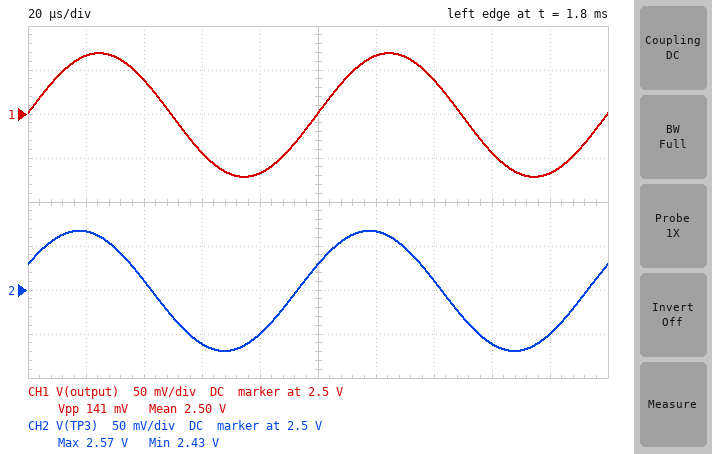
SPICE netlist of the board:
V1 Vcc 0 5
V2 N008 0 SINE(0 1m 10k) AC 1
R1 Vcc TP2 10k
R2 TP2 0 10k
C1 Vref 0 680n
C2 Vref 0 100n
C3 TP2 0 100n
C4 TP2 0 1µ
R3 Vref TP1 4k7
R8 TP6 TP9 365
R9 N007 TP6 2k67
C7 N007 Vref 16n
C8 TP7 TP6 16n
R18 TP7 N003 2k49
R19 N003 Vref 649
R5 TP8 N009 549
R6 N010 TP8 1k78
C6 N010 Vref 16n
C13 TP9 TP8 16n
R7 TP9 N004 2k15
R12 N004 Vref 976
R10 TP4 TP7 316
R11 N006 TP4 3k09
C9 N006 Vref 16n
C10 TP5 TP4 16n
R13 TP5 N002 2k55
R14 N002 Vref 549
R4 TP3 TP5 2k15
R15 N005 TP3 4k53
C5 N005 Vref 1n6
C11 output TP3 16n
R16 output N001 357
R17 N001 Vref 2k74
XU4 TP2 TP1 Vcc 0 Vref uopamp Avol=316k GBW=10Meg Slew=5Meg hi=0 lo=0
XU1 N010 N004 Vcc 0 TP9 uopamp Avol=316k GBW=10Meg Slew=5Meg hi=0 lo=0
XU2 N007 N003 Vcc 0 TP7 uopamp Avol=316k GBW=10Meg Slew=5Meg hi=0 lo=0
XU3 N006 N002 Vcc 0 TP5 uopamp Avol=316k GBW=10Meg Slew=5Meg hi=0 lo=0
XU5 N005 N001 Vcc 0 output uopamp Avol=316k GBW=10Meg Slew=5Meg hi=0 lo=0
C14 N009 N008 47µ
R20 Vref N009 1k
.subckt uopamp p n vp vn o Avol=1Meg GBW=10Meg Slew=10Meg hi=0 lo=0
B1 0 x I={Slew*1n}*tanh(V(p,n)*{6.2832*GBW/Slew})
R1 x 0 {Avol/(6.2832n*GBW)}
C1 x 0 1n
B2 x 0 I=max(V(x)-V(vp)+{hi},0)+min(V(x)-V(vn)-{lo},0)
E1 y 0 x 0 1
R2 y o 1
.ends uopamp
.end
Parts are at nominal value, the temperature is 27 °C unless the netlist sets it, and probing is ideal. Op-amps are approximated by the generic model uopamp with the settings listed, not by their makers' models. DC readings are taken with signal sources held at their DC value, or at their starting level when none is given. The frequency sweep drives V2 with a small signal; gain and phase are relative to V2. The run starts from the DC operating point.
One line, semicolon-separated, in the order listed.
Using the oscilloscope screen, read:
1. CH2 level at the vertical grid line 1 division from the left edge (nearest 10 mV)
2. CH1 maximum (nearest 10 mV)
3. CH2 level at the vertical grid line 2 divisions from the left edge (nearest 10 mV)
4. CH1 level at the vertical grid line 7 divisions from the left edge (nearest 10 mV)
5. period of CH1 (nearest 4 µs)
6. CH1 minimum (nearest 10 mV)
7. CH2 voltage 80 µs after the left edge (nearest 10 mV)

2.57 V; 2.57 V; 2.51 V; 2.54 V; 100 µs; 2.43 V; 2.45 V
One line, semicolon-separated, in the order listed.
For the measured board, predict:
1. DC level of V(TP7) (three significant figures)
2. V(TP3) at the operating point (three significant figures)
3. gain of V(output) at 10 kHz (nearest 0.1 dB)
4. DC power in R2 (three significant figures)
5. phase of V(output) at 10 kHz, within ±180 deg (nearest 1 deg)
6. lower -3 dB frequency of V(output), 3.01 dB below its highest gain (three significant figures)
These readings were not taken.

2.50 V; 2.50 V; 36.9 dB; 625 µW; 2 deg; 3.39 Hz
